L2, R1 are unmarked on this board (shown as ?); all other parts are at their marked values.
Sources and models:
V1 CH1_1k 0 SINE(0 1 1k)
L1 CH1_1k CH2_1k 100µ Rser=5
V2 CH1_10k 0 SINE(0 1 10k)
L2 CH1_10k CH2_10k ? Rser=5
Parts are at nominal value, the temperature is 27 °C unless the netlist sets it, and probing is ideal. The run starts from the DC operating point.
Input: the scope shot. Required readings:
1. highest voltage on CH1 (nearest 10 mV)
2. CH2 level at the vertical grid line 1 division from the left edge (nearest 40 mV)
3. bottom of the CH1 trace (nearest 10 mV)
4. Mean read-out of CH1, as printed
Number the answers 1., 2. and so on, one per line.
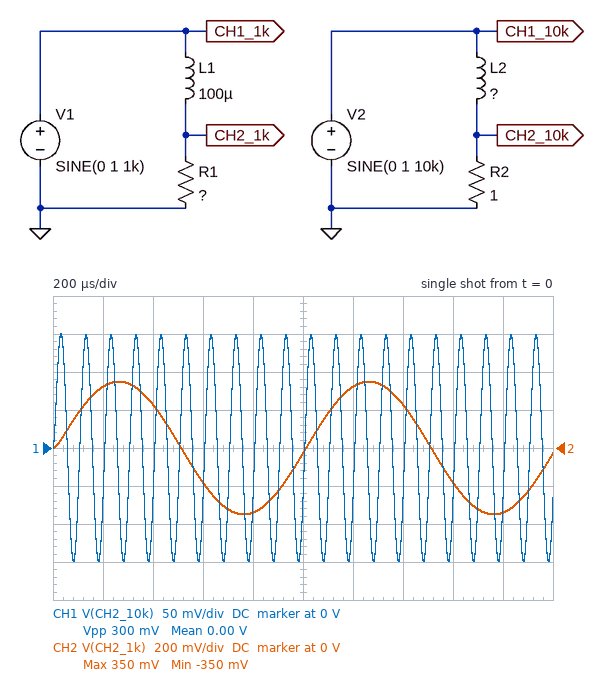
1. 150 mV
2. 320 mV
3. -150 mV
4. 0.00 V
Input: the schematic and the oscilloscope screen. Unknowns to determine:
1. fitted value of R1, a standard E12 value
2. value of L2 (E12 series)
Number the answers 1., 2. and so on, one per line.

1. 2.7 Ω
2. 47 µH
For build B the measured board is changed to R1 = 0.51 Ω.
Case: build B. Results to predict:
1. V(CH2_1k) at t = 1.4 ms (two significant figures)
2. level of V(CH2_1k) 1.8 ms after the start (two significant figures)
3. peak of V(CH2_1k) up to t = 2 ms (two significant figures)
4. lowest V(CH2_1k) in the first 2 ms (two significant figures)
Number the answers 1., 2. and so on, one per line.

1. 62 mV
2. -90 mV
3. 92 mV
4. -92 mV
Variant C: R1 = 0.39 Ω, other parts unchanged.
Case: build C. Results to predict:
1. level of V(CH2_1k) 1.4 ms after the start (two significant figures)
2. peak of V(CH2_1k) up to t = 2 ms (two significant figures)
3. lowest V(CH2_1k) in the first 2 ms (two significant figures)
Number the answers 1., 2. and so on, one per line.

1. 49 mV
2. 72 mV
3. -72 mV
